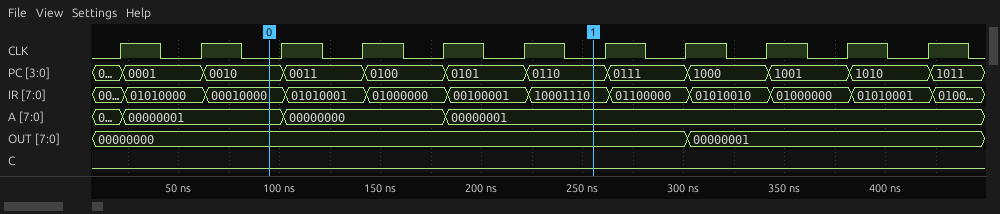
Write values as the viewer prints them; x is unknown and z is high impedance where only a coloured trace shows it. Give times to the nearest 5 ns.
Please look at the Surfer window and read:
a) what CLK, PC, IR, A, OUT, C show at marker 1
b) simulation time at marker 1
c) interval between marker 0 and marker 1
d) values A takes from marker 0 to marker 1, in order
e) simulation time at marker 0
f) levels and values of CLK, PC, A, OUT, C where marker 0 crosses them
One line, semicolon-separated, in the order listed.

CLK=0, PC=0110, IR=10001110, A=00000001, OUT=00000000, C=0; 255 ns; 160 ns; 00000001, 00000000, 00000001; 95 ns; CLK=0, PC=0010, A=00000001, OUT=00000000, C=0
